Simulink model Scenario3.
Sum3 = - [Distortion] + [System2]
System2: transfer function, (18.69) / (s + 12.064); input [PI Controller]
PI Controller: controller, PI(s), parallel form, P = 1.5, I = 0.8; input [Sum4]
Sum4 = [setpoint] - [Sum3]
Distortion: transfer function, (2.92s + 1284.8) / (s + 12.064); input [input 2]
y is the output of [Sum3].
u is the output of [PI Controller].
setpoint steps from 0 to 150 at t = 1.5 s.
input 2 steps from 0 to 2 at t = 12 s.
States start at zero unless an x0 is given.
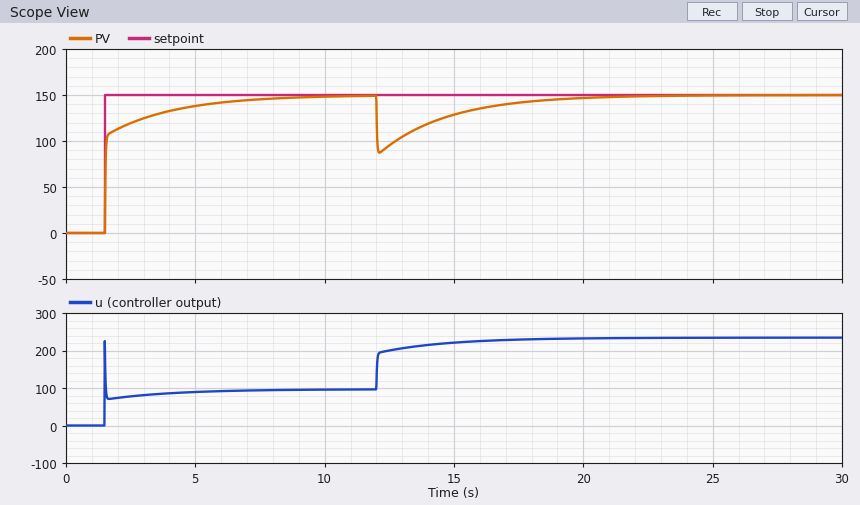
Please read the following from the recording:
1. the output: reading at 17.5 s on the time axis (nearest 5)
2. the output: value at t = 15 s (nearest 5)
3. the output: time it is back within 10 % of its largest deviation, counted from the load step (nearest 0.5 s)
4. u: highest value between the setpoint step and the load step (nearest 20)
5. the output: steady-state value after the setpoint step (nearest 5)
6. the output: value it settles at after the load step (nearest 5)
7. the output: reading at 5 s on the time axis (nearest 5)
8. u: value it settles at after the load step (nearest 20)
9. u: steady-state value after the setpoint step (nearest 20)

140
130
6.5 s
220
150
150
140
240
100
